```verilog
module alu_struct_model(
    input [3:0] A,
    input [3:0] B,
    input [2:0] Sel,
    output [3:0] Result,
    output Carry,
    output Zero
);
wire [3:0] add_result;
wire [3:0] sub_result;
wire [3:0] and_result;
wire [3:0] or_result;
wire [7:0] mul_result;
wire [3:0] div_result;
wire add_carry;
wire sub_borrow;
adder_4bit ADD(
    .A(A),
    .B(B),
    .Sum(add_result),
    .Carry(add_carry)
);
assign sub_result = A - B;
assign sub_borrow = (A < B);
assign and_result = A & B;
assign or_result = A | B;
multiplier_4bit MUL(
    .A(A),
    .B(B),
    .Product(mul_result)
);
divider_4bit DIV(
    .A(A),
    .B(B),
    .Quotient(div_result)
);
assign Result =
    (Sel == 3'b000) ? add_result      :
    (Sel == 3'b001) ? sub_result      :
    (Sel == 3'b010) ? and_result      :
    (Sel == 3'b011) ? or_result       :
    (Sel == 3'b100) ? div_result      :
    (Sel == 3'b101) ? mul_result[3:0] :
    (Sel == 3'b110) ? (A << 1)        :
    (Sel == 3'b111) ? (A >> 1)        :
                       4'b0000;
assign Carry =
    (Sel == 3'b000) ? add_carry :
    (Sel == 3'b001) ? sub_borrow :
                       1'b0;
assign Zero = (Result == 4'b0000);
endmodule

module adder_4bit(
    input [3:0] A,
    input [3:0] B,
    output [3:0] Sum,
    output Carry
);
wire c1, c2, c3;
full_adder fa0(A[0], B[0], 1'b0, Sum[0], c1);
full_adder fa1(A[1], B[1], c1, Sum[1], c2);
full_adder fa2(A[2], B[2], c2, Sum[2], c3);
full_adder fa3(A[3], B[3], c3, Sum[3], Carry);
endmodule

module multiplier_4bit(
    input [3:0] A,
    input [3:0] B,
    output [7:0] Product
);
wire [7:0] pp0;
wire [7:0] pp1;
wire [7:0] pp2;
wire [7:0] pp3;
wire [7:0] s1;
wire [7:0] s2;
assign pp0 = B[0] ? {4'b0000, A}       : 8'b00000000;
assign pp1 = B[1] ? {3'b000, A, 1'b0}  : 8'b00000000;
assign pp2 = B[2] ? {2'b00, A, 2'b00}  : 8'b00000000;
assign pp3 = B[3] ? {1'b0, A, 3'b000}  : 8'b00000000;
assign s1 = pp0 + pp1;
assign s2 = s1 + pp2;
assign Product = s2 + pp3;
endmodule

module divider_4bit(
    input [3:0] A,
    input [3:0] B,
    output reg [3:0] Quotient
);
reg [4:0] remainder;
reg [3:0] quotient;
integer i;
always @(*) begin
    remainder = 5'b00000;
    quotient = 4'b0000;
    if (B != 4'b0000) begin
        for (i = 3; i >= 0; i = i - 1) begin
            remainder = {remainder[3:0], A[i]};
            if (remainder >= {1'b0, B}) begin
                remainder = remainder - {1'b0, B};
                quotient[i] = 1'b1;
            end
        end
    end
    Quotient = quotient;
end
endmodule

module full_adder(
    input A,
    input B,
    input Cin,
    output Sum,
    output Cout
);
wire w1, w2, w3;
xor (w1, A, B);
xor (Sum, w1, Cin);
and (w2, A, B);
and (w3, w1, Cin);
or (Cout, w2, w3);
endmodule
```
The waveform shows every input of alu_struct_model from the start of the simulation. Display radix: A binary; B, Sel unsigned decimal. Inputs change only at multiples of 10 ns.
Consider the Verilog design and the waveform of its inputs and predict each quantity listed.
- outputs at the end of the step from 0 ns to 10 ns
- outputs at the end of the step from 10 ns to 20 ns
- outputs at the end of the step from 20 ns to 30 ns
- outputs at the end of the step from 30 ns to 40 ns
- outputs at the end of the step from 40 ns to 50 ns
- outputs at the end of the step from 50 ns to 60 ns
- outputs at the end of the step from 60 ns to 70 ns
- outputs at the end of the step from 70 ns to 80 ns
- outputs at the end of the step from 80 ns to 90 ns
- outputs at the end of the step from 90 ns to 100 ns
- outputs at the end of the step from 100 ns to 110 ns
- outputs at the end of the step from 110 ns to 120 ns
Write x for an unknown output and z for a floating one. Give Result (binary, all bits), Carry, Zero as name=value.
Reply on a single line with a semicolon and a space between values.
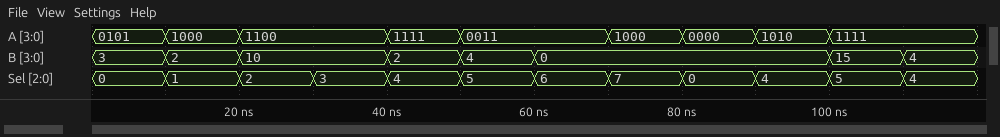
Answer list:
Result=1000, Carry=0, Zero=0; Result=0110, Carry=0, Zero=0; Result=1000, Carry=0, Zero=0; Result=1110, Carry=0, Zero=0; Result=0111, Carry=0, Zero=0; Result=1100, Carry=0, Zero=0; Result=0110, Carry=0, Zero=0; Result=0100, Carry=0, Zero=0; Result=0000, Carry=0, Zero=1; Result=0000, Carry=0, Zero=1; Result=0001, Carry=0, Zero=0; Result=0011, Carry=0, Zero=0
